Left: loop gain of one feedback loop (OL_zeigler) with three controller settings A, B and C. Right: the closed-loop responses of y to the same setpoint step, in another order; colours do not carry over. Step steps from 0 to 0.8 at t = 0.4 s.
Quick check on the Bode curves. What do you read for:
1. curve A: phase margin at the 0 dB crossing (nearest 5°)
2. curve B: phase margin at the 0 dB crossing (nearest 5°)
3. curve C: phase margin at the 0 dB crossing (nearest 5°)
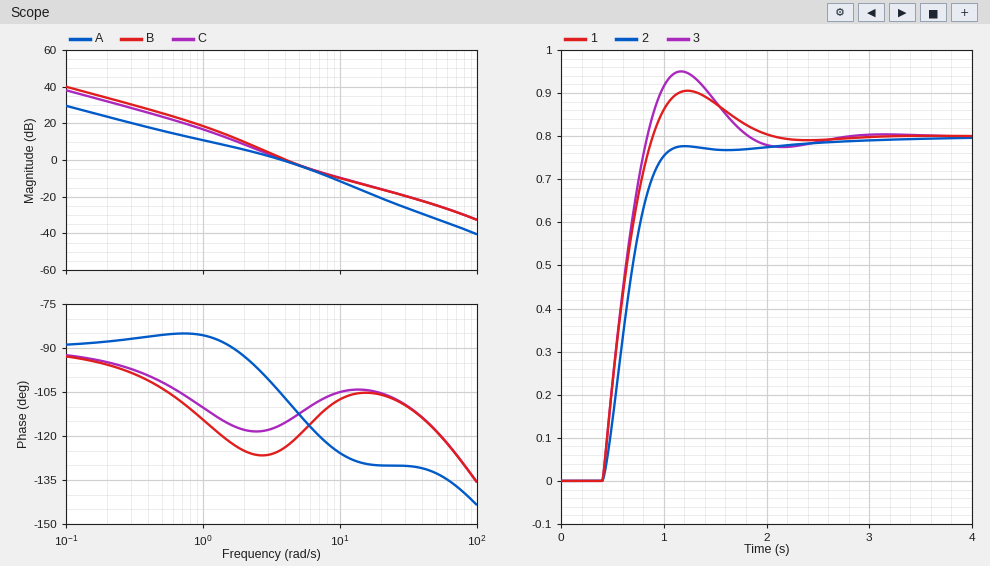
75°
55°
65°
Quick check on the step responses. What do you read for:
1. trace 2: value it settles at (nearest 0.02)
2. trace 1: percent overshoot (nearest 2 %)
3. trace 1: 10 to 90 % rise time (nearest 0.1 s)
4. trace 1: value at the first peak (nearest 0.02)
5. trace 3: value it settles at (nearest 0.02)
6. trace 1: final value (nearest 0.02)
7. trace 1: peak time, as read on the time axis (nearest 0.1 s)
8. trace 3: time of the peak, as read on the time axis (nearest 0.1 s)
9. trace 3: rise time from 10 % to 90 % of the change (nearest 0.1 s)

0.80
14 %
0.4 s
0.90
0.80
0.80
1.2 s
1.2 s
0.3 s
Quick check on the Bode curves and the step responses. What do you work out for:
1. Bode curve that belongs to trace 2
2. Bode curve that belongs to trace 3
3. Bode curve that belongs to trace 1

A
B
C
